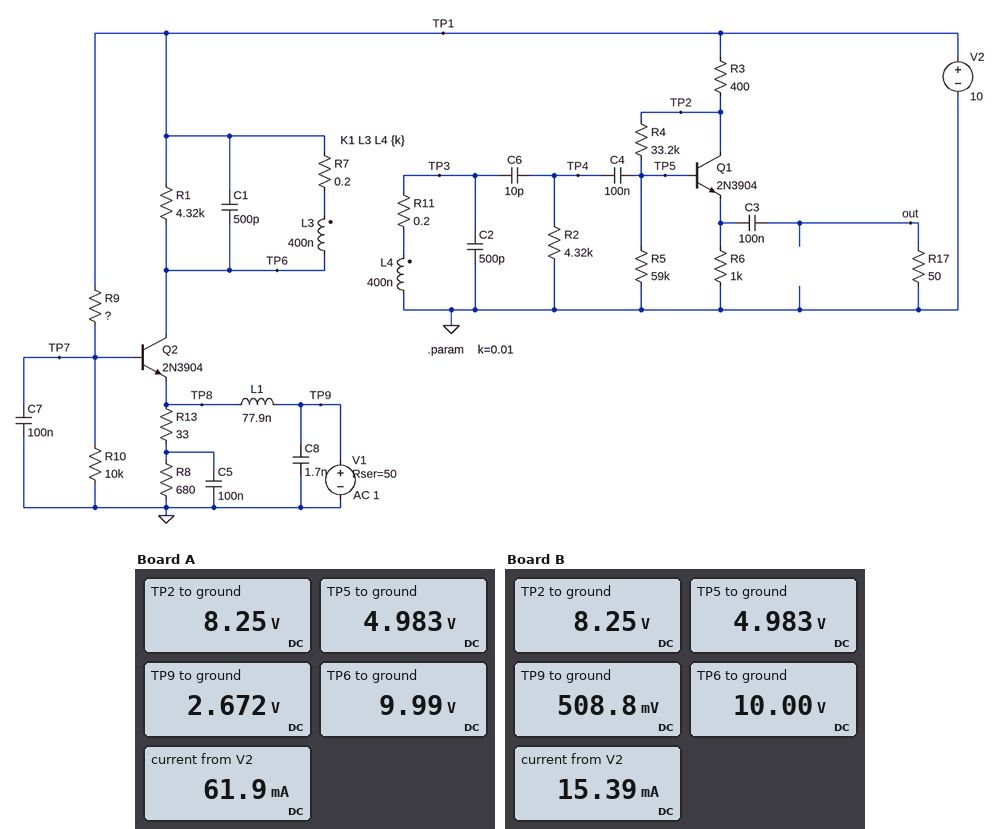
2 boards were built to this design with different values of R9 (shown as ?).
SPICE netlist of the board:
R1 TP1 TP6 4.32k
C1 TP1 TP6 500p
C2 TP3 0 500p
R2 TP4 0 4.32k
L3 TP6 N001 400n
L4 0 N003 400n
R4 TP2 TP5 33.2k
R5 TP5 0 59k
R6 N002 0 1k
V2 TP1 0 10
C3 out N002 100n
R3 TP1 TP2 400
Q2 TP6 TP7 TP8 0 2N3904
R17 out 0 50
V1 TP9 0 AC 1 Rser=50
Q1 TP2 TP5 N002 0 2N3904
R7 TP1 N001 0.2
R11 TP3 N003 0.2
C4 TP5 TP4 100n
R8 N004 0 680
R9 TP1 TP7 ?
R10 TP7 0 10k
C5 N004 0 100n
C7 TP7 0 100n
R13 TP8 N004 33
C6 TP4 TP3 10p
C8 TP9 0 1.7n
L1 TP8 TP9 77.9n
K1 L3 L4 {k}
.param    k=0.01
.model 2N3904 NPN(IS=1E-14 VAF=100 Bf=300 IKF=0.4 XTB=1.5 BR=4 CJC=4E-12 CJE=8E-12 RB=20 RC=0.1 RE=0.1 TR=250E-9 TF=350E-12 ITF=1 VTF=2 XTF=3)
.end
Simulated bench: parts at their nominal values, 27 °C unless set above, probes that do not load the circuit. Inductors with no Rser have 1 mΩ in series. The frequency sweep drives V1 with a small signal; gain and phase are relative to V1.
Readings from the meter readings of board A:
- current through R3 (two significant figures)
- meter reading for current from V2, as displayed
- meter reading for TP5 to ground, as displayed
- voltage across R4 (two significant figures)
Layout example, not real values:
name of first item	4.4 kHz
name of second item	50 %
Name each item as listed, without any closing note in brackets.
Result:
current through R3	4.4 mA
meter reading for current from V2, as displayed	61.9 mA
meter reading for TP5 to ground, as displayed	4.983 V
voltage across R4	3.3 V
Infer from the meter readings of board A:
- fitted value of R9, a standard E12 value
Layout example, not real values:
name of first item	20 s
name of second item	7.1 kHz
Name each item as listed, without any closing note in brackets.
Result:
fitted value of R9, a standard E12 value	12 kΩ
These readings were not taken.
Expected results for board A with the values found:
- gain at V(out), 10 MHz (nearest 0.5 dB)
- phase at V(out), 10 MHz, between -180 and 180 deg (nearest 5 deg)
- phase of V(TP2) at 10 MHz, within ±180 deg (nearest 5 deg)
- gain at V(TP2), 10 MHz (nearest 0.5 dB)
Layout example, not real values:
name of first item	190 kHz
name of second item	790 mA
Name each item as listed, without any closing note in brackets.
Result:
gain at V(out), 10 MHz	-24.5 dB
phase at V(out), 10 MHz, between -180 and 180 deg	-100 deg
phase of V(TP2) at 10 MHz, within ±180 deg	75 deg
gain at V(TP2), 10 MHz	-6.0 dB
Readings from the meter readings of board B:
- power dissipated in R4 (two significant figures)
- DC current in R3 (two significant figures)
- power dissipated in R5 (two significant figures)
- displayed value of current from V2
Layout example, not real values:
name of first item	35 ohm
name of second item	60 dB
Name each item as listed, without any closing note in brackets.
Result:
power dissipated in R4	320 µW
DC current in R3	4.4 mA
power dissipated in R5	420 µW
displayed value of current from V2	15.39 mA
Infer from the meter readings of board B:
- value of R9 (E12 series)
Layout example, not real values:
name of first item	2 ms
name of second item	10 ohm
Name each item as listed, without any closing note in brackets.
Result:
value of R9	56 kΩ
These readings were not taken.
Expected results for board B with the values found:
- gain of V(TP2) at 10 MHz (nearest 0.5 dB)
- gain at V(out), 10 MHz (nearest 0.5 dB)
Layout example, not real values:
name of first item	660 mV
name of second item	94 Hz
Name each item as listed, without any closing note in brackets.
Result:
gain of V(TP2) at 10 MHz	-8.5 dB
gain at V(out), 10 MHz	-27.0 dB
